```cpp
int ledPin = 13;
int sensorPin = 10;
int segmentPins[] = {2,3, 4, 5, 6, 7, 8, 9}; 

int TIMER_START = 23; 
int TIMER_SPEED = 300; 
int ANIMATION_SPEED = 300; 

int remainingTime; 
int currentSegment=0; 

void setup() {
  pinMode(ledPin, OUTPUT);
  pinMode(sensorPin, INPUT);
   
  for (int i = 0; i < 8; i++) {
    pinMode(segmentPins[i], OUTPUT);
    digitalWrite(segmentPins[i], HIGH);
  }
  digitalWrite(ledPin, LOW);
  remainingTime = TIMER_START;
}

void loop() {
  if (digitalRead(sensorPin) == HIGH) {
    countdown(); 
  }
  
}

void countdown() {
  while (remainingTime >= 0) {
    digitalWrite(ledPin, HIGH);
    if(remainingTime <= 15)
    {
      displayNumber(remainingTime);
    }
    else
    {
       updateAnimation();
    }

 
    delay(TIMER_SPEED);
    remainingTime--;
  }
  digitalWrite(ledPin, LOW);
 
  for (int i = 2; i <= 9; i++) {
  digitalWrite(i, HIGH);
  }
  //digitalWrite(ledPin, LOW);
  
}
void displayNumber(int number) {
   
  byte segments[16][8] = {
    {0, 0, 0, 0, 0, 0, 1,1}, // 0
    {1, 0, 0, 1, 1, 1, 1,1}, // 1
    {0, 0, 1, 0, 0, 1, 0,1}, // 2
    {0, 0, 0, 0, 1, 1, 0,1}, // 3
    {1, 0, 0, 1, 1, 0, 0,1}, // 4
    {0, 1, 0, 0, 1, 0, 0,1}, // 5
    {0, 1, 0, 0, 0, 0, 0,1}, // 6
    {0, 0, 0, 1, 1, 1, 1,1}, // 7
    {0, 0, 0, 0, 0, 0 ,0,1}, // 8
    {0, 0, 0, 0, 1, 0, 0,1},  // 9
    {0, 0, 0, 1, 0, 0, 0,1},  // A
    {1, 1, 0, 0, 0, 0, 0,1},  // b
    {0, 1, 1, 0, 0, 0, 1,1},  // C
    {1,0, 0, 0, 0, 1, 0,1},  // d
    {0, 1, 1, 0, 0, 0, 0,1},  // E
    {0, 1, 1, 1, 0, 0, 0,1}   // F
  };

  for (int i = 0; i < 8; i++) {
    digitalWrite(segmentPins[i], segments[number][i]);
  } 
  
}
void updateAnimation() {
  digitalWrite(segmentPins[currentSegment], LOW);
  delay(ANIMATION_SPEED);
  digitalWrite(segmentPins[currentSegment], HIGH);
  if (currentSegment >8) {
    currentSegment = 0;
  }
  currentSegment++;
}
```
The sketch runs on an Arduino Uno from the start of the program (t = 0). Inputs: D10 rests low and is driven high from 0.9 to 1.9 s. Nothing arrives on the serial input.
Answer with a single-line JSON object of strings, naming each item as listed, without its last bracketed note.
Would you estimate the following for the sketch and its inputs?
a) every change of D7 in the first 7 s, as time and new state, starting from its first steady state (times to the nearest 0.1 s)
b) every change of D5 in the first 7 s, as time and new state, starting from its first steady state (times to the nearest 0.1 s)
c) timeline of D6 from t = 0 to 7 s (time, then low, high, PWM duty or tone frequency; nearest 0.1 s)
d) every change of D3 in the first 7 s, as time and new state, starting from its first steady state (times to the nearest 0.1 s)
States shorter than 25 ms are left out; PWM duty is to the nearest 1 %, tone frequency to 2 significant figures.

{"every change of D7 in the first 7 s, as time and new state, starting from its first steady state": "0 s high; 3.9 s low; 4.2 s high; 5.7 s low; 6.3 s high; 6.6 s low", "every change of D5 in the first 7 s, as time and new state, starting from its first steady state": "0 s high; 2.7 s low; 3 s high; 6 s low", "timeline of D6 from t = 0 to 7 s": "0 s high; 3.3 s low; 3.6 s high; 5.7 s low", "every change of D3 in the first 7 s, as time and new state, starting from its first steady state": "0 s high; 1.5 s low; 1.8 s high; 6.3 s low; 6.6 s high"}
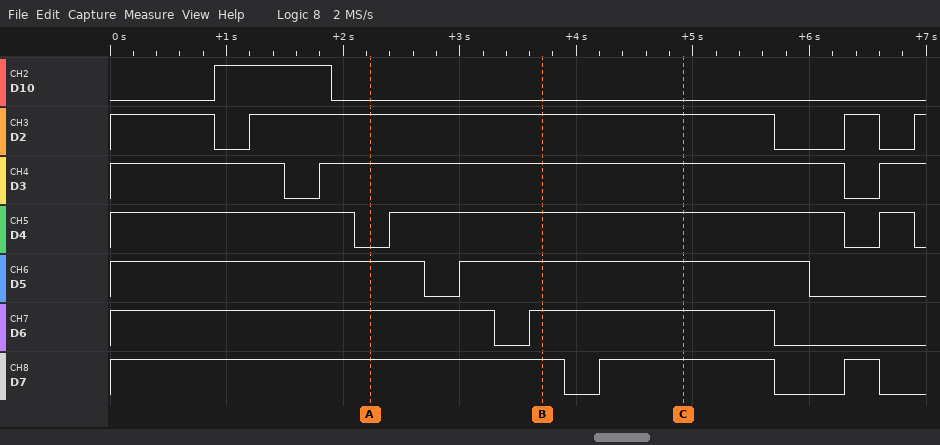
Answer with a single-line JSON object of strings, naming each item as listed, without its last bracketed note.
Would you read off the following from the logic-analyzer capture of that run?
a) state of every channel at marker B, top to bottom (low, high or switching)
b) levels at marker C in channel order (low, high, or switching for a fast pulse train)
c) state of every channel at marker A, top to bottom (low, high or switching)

{"state of every channel at marker B, top to bottom": "D10 low, D2 high, D3 high, D4 high, D5 high, D6 high, D7 high", "levels at marker C in channel order": "D10 low, D2 high, D3 high, D4 high, D5 high, D6 high, D7 high", "state of every channel at marker A, top to bottom": "D10 low, D2 high, D3 high, D4 low, D5 high, D6 high, D7 high"}
